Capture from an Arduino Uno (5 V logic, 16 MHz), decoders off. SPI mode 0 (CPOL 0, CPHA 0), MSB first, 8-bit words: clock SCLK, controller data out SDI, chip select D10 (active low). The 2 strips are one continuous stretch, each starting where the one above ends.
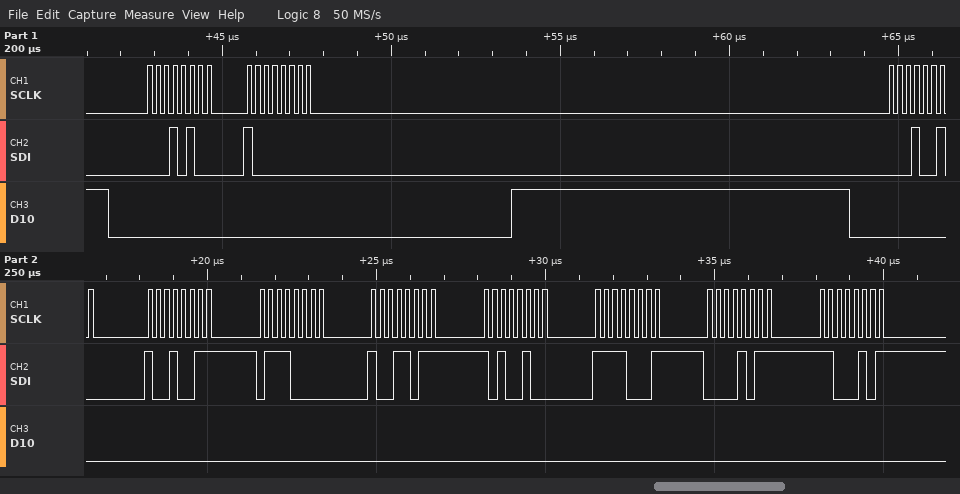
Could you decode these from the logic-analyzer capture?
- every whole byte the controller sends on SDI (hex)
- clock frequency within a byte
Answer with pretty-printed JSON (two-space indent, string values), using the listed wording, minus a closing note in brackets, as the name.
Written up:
{
  "every whole byte the controller sends on SDI": "14 80 12 93 70 9B A4 F1 0B C5",
  "clock frequency within a byte": "4 MHz"
}
